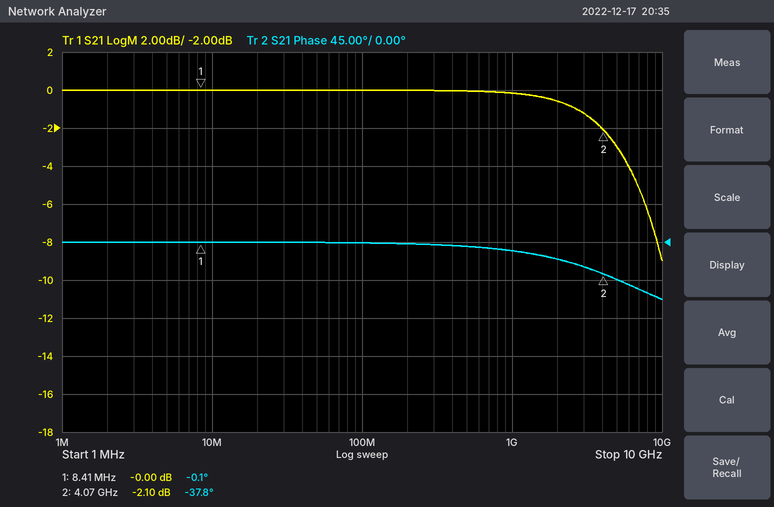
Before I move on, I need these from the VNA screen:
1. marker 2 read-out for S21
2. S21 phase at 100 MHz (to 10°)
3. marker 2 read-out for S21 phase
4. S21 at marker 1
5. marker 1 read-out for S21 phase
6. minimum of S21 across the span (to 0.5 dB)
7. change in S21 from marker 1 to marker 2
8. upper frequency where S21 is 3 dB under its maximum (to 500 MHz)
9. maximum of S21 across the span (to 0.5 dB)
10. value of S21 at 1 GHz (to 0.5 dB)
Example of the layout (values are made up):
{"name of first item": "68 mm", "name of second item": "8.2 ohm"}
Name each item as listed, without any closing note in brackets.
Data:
{"marker 2 read-out for S21": "-2.10 dB", "S21 phase at 100 MHz": "0°", "marker 2 read-out for S21 phase": "-37.8°", "S21 at marker 1": "-0.00 dB", "marker 1 read-out for S21 phase": "-0.1°", "minimum of S21 across the span": "-9.0 dB", "change in S21 from marker 1 to marker 2": "-2.10 dB", "upper frequency where S21 is 3 dB under its maximum": "5.0 GHz", "maximum of S21 across the span": "0.0 dB", "value of S21 at 1 GHz": "0.0 dB"}
